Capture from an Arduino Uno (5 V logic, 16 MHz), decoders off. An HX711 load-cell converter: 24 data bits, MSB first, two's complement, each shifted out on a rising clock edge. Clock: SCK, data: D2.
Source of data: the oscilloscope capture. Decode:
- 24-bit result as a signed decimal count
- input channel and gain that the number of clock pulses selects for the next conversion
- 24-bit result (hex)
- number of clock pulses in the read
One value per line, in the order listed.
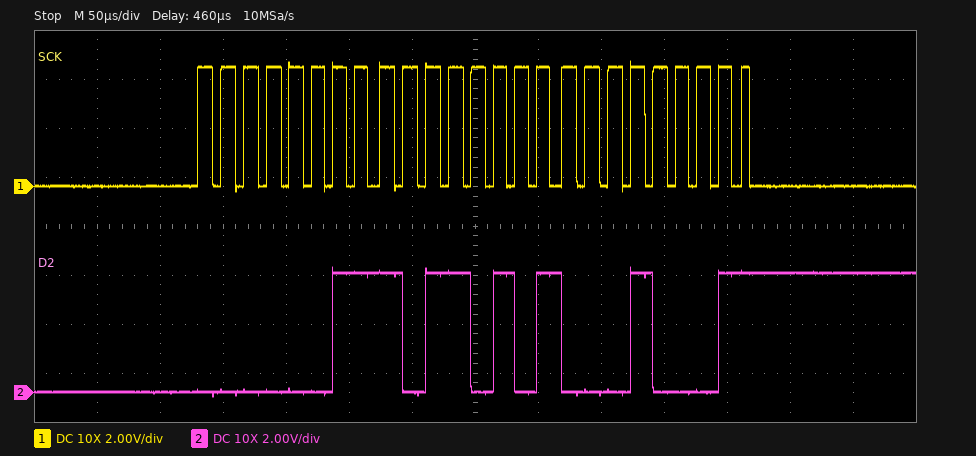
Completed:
242961
channel A, gain 128
0x03B511
25
